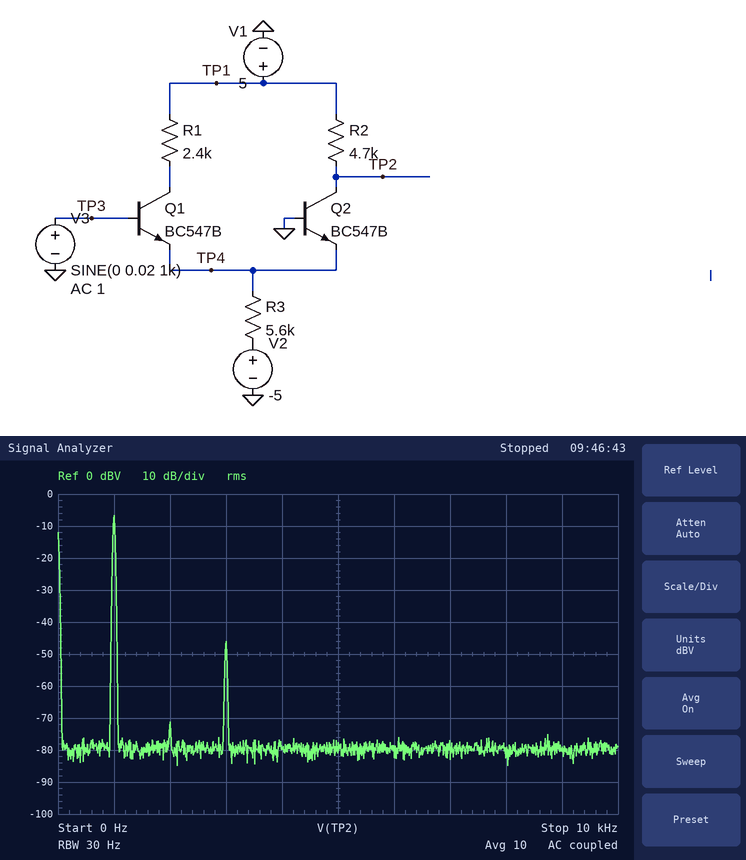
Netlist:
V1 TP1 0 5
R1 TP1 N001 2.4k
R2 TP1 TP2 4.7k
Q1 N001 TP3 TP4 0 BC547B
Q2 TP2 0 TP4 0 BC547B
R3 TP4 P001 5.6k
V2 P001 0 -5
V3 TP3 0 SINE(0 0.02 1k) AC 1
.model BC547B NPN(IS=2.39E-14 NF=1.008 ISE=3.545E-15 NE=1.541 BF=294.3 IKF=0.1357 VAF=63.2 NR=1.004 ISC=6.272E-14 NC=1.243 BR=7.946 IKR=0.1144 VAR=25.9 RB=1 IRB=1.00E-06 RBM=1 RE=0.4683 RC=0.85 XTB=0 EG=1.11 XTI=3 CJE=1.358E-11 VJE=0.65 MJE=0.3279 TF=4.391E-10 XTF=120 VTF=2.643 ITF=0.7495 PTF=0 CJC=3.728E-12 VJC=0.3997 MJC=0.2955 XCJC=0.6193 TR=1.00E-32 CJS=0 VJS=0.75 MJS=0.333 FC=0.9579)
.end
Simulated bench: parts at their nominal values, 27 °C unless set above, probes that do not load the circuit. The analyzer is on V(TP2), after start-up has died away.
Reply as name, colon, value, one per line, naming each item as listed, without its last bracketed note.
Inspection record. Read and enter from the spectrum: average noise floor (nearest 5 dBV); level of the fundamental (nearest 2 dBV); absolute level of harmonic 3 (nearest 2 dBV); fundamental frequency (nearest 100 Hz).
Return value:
average noise floor: -80 dBV
level of the fundamental: -6 dBV
absolute level of harmonic 3: -46 dBV
fundamental frequency: 1.0 kHz
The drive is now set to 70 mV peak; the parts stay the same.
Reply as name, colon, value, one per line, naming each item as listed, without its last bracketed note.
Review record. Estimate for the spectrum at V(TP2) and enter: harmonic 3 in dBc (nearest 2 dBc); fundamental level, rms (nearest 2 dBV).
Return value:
harmonic 3 in dBc: -20 dBc
fundamental level, rms: 2 dBV
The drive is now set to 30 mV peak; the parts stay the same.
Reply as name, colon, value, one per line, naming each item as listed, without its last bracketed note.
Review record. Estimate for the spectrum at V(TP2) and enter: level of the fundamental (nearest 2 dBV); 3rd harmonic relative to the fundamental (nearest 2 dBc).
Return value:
level of the fundamental: -4 dBV
3rd harmonic relative to the fundamental: -32 dBc
